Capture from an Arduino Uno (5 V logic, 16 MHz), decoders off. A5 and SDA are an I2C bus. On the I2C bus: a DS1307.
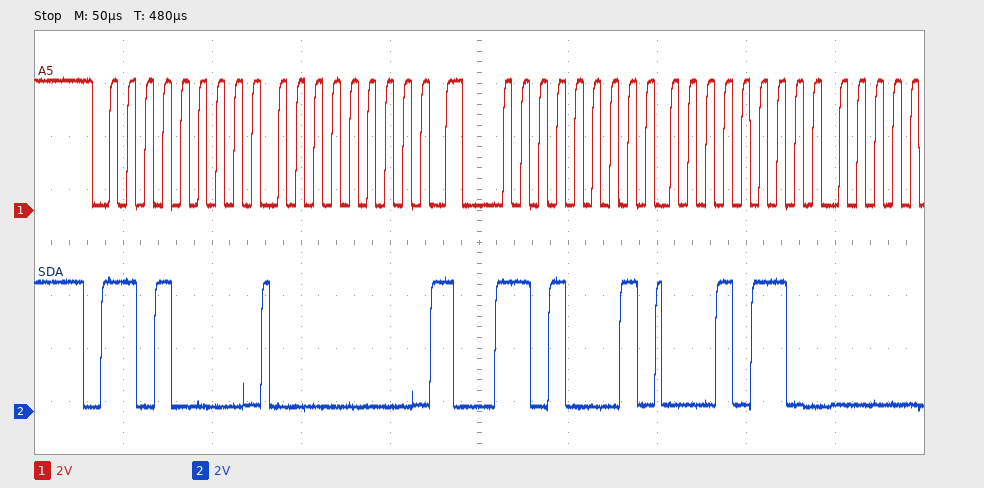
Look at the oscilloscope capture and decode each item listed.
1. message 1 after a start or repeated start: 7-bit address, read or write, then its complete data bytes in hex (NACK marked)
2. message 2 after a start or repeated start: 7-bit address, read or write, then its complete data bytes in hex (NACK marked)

0x68 write: 00
0x68 read: 16
